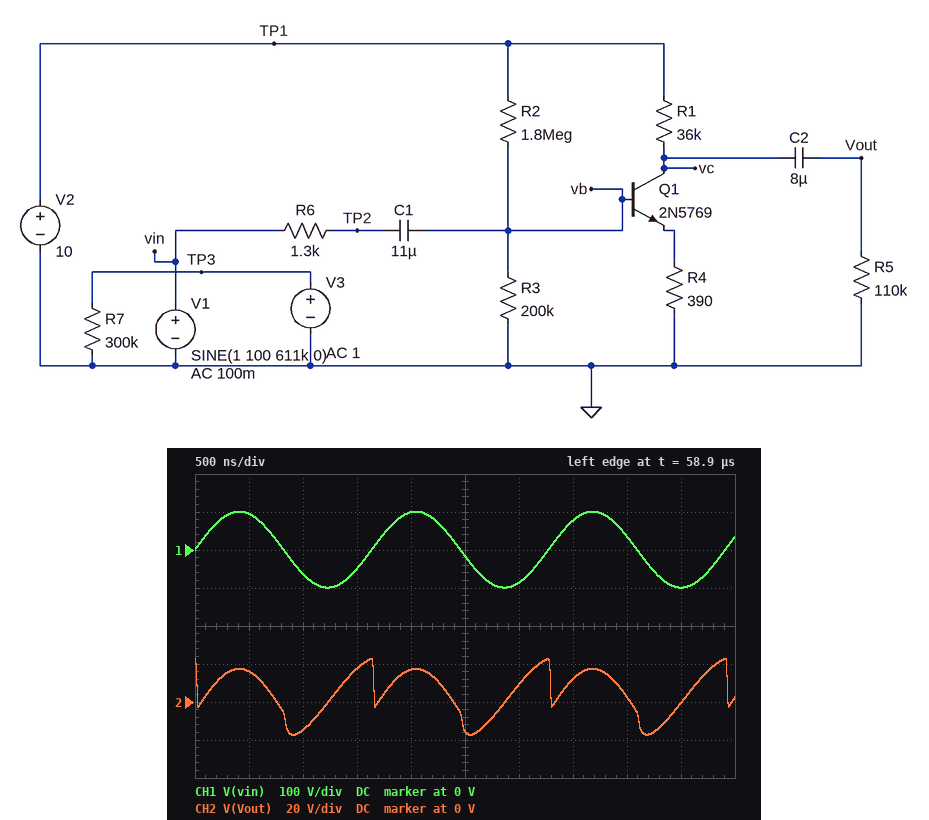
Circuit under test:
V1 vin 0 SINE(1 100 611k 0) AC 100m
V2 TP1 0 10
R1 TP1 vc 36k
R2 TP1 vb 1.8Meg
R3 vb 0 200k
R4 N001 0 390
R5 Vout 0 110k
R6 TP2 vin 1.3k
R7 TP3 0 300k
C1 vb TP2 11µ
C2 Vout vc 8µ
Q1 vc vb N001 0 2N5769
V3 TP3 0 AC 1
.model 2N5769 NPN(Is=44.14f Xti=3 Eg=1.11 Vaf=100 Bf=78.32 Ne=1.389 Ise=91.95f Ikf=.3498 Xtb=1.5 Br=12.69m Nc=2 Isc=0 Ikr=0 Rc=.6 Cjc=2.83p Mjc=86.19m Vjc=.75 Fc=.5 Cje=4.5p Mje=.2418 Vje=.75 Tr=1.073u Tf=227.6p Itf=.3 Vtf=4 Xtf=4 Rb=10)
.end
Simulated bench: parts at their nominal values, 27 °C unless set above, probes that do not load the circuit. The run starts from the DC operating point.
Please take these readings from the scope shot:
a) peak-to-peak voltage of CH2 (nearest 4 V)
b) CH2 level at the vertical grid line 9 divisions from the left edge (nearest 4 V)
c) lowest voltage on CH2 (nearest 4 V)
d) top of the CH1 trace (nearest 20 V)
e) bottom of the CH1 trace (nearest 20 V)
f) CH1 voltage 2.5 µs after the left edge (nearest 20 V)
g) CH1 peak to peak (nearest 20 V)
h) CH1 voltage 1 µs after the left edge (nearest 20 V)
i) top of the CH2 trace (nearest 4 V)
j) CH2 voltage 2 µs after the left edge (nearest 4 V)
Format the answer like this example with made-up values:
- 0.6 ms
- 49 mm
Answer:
- 40 V
- 0 V
- -16 V
- 100 V
- -100 V
- -20 V
- 200 V
- -60 V
- 24 V
- 16 V
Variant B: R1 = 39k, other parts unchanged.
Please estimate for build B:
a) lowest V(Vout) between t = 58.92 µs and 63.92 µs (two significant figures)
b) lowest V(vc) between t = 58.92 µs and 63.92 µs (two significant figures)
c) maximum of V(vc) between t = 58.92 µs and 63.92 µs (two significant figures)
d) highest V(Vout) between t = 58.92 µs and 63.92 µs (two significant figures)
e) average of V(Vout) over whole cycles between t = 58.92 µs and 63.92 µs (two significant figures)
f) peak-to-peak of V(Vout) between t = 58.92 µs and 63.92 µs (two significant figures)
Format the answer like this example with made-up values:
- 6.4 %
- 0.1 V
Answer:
- -18 V
- -13 V
- 29 V
- 24 V
- 5.5 V
- 42 V
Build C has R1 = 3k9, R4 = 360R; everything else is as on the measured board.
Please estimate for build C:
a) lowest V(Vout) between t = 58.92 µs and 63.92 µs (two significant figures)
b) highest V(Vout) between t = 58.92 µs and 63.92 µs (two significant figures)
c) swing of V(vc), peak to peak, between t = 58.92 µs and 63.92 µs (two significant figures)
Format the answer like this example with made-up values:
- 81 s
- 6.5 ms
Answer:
- -9.6 V
- 11 V
- 21 V
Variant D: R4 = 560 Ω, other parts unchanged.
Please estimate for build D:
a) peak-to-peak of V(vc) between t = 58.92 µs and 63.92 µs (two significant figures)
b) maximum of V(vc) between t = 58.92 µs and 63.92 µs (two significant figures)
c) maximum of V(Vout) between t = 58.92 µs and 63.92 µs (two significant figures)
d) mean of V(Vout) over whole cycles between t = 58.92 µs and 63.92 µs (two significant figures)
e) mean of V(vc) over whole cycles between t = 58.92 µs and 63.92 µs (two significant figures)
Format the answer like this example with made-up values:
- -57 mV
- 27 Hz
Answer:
- 41 V
- 30 V
- 24 V
- 7.3 V
- 13 V
